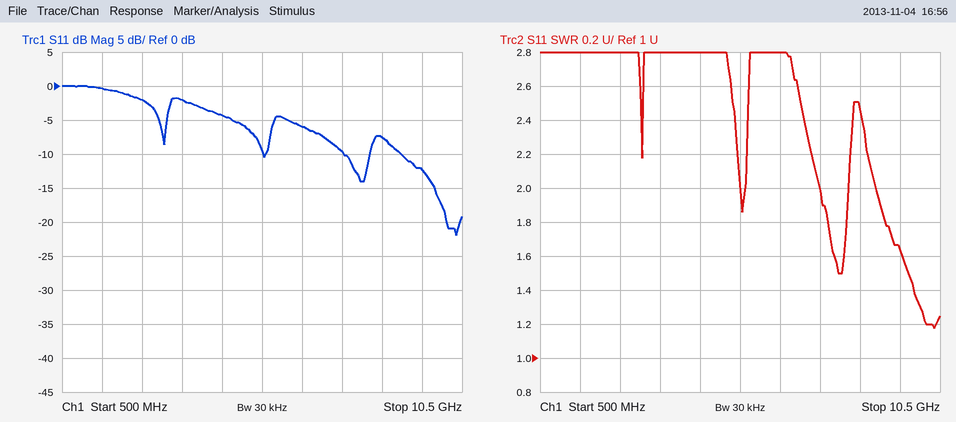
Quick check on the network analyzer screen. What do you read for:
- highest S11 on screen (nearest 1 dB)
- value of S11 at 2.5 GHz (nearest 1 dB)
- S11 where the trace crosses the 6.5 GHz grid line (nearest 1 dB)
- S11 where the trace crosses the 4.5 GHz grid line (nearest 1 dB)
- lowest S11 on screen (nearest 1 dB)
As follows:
0 dB
-2 dB
-6 dB
-4 dB
-22 dB
